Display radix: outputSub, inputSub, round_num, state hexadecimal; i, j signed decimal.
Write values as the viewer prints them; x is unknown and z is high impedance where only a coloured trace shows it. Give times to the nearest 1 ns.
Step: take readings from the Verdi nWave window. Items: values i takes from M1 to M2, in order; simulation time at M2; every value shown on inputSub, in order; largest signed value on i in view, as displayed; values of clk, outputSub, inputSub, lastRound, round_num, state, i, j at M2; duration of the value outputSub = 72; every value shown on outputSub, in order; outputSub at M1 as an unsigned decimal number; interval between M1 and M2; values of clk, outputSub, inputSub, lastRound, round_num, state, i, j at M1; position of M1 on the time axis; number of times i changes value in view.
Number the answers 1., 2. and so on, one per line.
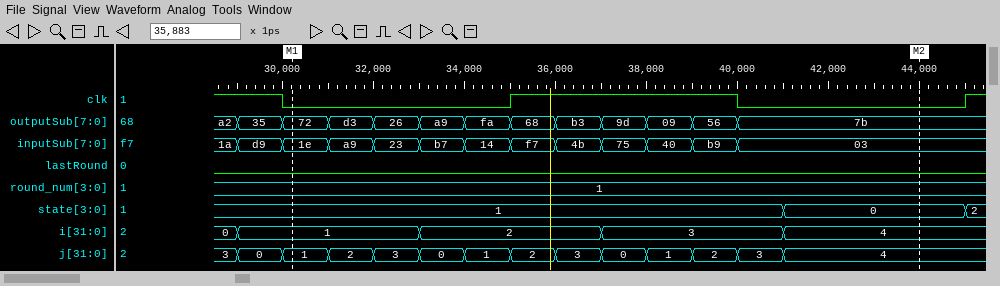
1. 1, 2, 3, 4
2. 44 ns
3. 1a, d9, 1e, a9, 23, b7, 14, f7, 4b, 75, 40, b9, 03
4. 4
5. clk=0, outputSub=7b, inputSub=03, lastRound=0, round_num=1, state=0, i=4, j=4
6. 1 ns
7. a2, 35, 72, d3, 26, a9, fa, 68, b3, 9d, 09, 56, 7b
8. 114
9. 14 ns
10. clk=0, outputSub=72, inputSub=1e, lastRound=0, round_num=1, state=1, i=1, j=1
11. 30 ns
12. 4
